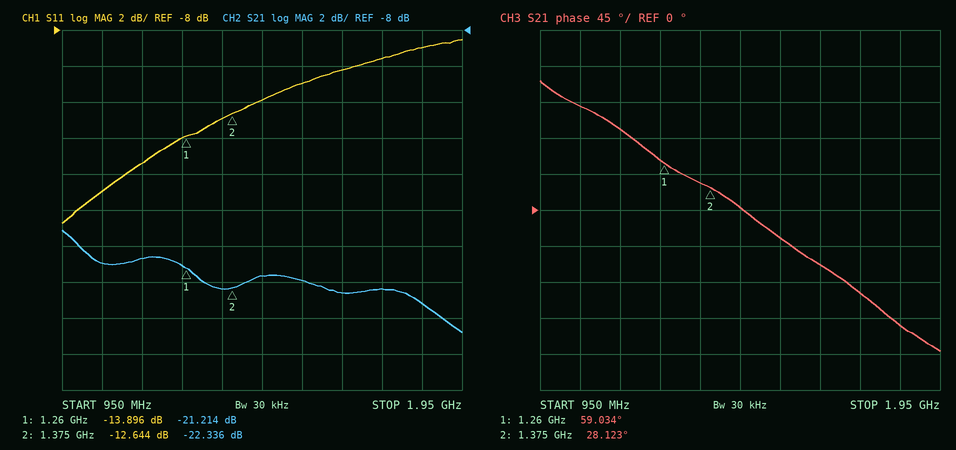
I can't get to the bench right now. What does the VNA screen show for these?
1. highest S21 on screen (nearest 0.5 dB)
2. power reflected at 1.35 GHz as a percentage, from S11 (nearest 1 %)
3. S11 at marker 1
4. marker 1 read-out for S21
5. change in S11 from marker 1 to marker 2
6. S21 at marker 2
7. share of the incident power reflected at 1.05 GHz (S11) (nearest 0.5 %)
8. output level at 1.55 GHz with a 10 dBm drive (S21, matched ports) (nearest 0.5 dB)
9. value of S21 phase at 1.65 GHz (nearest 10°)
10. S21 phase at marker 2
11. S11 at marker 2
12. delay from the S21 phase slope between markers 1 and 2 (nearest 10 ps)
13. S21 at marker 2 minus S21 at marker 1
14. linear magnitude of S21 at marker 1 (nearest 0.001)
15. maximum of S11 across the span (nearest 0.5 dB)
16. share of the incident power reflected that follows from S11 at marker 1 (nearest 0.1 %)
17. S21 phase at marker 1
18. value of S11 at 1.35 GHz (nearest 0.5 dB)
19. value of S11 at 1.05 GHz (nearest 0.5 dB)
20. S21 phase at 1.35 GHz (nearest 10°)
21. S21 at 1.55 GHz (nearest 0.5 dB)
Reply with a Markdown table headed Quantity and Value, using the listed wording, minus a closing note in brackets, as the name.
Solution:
| Quantity | Value |
|---|---|
| highest S21 on screen | -19.0 dB |
| power reflected at 1.35 GHz as a percentage, from S11 | 5 % |
| S11 at marker 1 | -13.896 dB |
| marker 1 read-out for S21 | -21.214 dB |
| change in S11 from marker 1 to marker 2 | 1.252 dB |
| S21 at marker 2 | -22.336 dB |
| share of the incident power reflected at 1.05 GHz (S11) | 2.0 % |
| output level at 1.55 GHz with a 10 dBm drive (S21, matched ports) | -12.0 dBm |
| value of S21 phase at 1.65 GHz | -70° |
| S21 phase at marker 2 | 28.123° |
| S11 at marker 2 | -12.644 dB |
| delay from the S21 phase slope between markers 1 and 2 | 750 ps |
| S21 at marker 2 minus S21 at marker 1 | -1.122 dB |
| linear magnitude of S21 at marker 1 | 0.087 |
| maximum of S11 across the span | -8.5 dB |
| share of the incident power reflected that follows from S11 at marker 1 | 4.1 % |
| S21 phase at marker 1 | 59.034° |
| value of S11 at 1.35 GHz | -13.0 dB |
| value of S11 at 1.05 GHz | -17.0 dB |
| S21 phase at 1.35 GHz | 30° |
| S21 at 1.55 GHz | -22.0 dB |
